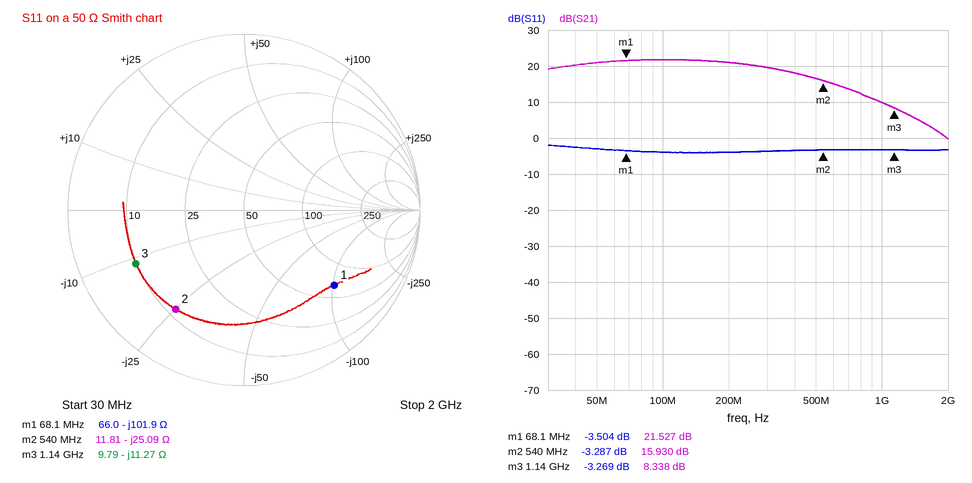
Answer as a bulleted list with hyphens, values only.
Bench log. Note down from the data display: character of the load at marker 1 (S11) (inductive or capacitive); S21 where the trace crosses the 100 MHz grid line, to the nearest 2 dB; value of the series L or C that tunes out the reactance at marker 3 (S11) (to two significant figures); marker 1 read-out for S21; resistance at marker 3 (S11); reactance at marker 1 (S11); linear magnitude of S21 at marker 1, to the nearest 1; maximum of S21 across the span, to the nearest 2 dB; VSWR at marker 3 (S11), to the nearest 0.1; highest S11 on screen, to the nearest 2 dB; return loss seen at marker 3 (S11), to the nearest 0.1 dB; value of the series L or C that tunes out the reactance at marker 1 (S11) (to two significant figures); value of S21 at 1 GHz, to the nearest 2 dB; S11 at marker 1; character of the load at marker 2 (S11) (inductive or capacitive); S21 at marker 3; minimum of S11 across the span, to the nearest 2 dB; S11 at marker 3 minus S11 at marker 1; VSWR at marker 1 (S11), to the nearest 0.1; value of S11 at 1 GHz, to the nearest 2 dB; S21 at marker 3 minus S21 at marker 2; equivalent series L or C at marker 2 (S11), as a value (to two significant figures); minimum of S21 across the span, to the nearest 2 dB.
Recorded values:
- capacitive
- 22 dB
- 1.6 nH
- 21.527 dB
- 9.79 Ω
- -101.9 Ω
- 12
- 22 dB
- 5.4
- -2 dB
- 3.3 dB
- 240 nH
- 10 dB
- -3.504 dB
- capacitive
- 8.338 dB
- -4 dB
- 0.235 dB
- 5.0
- -4 dB
- -7.592 dB
- 12 pF
- 0 dB
